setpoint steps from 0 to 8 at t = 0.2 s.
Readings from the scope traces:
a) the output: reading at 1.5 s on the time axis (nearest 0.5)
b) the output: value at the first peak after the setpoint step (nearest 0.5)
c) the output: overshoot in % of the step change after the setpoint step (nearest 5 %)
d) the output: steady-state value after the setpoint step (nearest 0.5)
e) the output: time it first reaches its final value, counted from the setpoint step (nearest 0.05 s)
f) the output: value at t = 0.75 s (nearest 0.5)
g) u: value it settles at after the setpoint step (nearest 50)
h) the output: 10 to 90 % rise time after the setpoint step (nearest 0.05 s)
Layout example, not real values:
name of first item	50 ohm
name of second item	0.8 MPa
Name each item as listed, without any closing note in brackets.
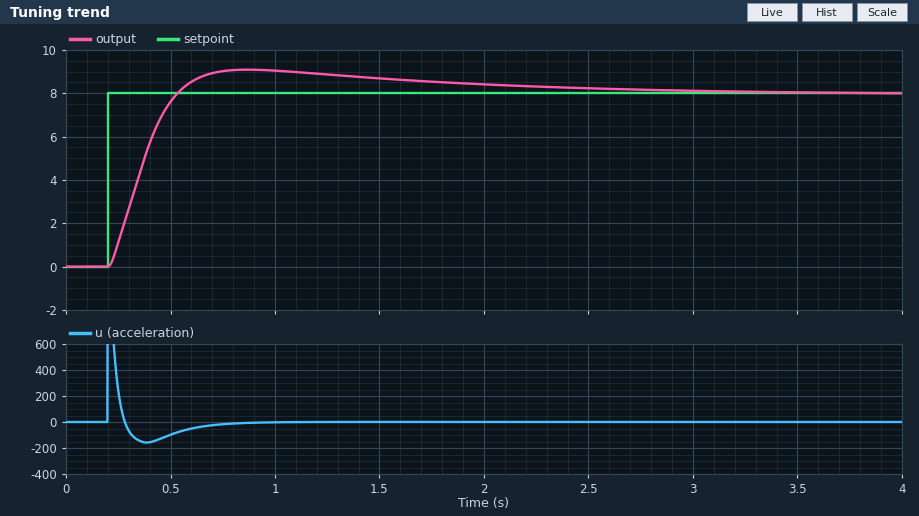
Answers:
the output: reading at 1.5 s on the time axis	8.5
the output: value at the first peak after the setpoint step	9.0
the output: overshoot in % of the step change after the setpoint step	15 %
the output: steady-state value after the setpoint step	8.0
the output: time it first reaches its final value, counted from the setpoint step	0.35 s
the output: value at t = 0.75 s	9.0
u: value it settles at after the setpoint step	0
the output: 10 to 90 % rise time after the setpoint step	0.25 s
